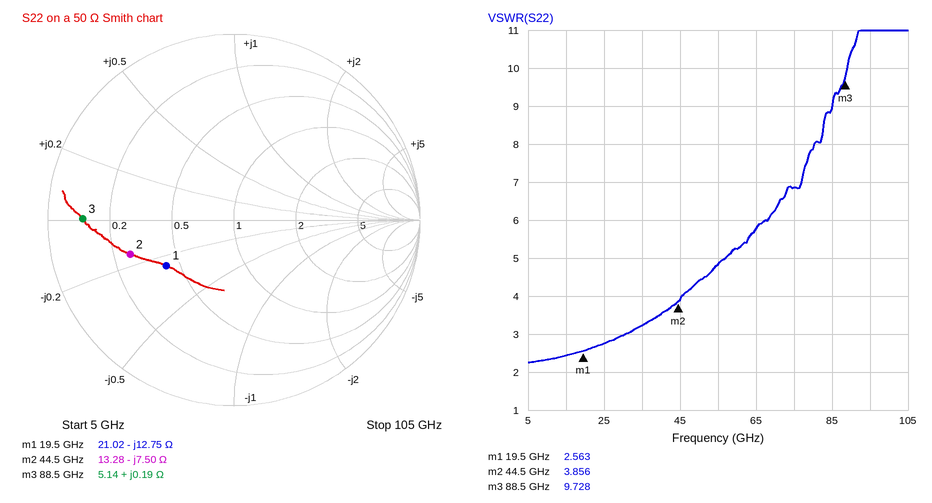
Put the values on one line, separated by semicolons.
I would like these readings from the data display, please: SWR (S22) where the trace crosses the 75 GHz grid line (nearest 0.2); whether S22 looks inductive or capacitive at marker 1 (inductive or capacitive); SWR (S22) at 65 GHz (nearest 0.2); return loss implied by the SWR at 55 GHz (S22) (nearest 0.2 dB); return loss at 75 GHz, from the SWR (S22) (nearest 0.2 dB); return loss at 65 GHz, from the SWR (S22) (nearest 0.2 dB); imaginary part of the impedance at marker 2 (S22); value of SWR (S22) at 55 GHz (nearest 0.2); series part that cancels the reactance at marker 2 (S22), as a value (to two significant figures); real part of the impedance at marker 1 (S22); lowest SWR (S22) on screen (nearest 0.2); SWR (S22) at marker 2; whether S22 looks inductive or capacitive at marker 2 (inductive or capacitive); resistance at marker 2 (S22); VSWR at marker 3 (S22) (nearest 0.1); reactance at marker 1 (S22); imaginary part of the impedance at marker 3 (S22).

6.8; capacitive; 5.8; 3.6 dB; 2.6 dB; 3.0 dB; -7.50 Ω; 4.8; 27 pH; 21.02 Ω; 2.2; 3.856; capacitive; 13.28 Ω; 9.7; -12.75 Ω; +0.19 Ω
